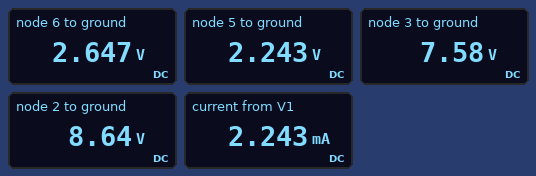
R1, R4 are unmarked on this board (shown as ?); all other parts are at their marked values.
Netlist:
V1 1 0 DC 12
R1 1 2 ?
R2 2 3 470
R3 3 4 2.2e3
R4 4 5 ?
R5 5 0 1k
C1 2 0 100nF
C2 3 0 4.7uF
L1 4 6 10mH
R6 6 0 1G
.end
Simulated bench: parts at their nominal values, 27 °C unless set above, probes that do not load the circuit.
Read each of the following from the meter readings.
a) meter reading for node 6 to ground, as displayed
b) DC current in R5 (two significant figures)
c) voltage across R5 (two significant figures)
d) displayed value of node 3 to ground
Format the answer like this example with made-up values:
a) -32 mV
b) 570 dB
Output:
a) 2.647 V
b) 2.2 mA
c) 2.2 V
d) 7.58 V
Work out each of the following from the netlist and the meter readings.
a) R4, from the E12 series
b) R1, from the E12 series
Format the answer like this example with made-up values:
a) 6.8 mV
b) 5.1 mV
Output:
a) 180 Ω
b) 1.5 kΩ
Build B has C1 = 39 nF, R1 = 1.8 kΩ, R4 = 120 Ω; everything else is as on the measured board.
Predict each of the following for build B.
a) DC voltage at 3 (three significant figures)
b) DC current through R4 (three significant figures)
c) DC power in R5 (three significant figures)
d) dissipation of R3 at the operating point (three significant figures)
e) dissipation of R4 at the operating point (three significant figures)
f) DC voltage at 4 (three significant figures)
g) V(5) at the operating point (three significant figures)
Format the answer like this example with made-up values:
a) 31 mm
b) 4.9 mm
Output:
a) 7.13 V
b) 2.15 mA
c) 4.61 mW
d) 10.1 mW
e) 553 µW
f) 2.40 V
g) 2.15 V
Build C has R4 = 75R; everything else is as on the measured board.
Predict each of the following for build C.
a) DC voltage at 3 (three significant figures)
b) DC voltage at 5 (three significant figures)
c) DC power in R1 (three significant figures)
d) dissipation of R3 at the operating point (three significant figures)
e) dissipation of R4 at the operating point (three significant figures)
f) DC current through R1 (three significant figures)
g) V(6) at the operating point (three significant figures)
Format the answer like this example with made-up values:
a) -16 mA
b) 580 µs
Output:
a) 7.49 V
b) 2.29 V
c) 7.85 mW
d) 11.5 mW
e) 393 µW
f) 2.29 mA
g) 2.46 V
